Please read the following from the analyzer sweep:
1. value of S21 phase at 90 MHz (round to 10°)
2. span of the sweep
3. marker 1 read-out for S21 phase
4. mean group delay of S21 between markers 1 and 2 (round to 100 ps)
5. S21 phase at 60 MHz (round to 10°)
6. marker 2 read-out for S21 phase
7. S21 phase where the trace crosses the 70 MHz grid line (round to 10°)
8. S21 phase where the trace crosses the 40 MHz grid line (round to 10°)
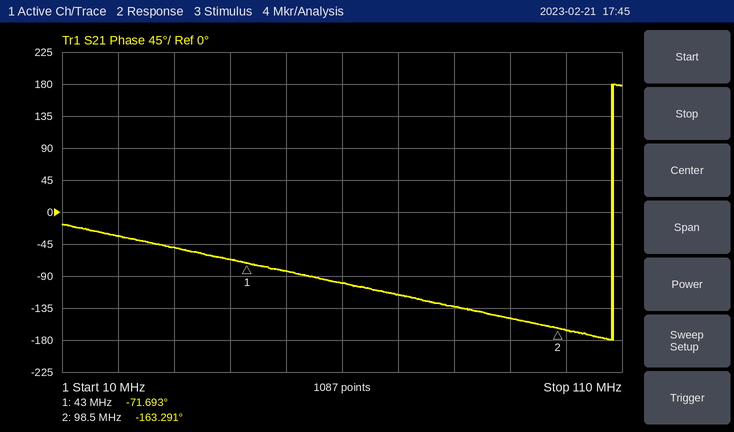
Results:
-150°
100 MHz
-71.693°
4.6 ns
-100°
-163.291°
-120°
-70°
